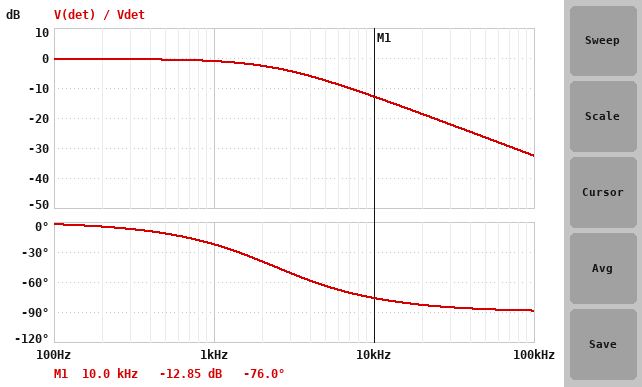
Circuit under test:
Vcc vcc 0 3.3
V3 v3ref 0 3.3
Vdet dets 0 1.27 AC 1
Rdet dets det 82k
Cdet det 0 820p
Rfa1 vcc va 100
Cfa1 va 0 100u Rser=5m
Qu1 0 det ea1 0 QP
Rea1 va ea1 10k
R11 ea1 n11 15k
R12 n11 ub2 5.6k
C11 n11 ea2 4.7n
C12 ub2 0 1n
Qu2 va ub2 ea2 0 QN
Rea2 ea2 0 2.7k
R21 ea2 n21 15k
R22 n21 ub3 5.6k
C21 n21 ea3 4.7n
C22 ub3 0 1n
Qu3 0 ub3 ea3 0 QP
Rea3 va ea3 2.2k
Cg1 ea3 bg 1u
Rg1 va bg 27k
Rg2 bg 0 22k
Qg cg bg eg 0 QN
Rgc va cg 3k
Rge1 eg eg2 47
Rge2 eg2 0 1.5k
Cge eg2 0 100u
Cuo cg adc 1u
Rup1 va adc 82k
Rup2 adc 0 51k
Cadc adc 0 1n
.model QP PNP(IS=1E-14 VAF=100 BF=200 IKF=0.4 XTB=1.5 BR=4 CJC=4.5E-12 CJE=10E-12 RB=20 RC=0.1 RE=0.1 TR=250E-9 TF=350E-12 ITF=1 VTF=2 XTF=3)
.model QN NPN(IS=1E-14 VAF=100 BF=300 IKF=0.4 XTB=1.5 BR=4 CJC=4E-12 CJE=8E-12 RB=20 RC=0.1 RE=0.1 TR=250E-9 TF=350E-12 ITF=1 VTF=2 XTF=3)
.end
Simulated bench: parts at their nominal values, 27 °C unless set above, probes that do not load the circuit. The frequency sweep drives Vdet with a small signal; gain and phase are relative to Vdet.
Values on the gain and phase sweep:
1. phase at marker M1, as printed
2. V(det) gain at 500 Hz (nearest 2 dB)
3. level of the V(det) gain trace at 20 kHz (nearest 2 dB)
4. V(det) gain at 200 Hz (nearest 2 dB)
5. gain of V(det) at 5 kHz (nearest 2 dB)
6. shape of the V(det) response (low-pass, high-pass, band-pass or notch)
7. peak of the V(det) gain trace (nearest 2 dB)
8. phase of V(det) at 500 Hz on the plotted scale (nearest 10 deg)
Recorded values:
-76.0 deg
0 dB
-18 dB
0 dB
-8 dB
low-pass
0 dB
-10 deg
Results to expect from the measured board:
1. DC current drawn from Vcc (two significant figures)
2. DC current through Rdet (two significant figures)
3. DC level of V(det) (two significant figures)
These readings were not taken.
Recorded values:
1.7 mA
590 nA
1.3 V
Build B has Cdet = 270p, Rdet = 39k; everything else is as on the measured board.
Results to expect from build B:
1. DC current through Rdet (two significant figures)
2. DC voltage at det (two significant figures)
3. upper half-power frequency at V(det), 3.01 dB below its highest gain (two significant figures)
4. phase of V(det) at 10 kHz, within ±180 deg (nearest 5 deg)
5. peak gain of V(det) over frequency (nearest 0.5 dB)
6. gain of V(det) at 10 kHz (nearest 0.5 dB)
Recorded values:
600 nA
1.3 V
15 kHz
-35 deg
0 dB
-2.0 dB
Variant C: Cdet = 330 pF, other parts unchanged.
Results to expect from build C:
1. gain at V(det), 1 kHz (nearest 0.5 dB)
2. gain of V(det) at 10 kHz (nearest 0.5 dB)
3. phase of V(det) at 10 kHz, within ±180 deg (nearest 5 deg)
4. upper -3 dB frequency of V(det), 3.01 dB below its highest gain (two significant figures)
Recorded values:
-0.5 dB
-6.0 dB
-60 deg
5.9 kHz
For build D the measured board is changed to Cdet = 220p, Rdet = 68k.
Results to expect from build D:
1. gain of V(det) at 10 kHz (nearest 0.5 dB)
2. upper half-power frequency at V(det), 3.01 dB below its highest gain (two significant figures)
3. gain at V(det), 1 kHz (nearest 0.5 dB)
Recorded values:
-3.0 dB
10 kHz
-0.5 dB
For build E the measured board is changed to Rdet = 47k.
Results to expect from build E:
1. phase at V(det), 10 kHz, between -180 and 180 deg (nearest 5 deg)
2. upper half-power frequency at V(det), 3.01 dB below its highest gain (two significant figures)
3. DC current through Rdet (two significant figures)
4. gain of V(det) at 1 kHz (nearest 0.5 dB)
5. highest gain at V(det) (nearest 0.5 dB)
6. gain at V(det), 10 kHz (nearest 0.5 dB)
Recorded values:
-65 deg
4.2 kHz
600 nA
-0.5 dB
0 dB
-8.5 dB
